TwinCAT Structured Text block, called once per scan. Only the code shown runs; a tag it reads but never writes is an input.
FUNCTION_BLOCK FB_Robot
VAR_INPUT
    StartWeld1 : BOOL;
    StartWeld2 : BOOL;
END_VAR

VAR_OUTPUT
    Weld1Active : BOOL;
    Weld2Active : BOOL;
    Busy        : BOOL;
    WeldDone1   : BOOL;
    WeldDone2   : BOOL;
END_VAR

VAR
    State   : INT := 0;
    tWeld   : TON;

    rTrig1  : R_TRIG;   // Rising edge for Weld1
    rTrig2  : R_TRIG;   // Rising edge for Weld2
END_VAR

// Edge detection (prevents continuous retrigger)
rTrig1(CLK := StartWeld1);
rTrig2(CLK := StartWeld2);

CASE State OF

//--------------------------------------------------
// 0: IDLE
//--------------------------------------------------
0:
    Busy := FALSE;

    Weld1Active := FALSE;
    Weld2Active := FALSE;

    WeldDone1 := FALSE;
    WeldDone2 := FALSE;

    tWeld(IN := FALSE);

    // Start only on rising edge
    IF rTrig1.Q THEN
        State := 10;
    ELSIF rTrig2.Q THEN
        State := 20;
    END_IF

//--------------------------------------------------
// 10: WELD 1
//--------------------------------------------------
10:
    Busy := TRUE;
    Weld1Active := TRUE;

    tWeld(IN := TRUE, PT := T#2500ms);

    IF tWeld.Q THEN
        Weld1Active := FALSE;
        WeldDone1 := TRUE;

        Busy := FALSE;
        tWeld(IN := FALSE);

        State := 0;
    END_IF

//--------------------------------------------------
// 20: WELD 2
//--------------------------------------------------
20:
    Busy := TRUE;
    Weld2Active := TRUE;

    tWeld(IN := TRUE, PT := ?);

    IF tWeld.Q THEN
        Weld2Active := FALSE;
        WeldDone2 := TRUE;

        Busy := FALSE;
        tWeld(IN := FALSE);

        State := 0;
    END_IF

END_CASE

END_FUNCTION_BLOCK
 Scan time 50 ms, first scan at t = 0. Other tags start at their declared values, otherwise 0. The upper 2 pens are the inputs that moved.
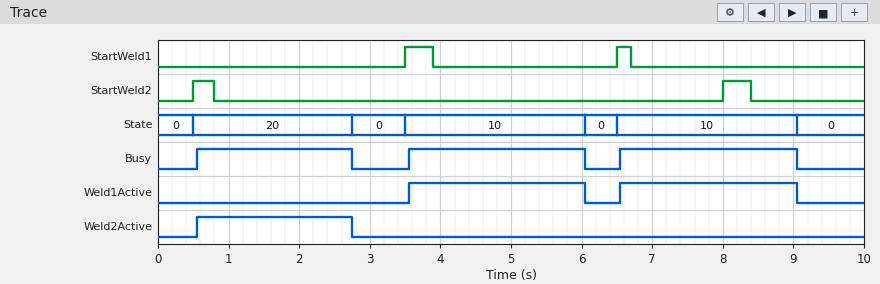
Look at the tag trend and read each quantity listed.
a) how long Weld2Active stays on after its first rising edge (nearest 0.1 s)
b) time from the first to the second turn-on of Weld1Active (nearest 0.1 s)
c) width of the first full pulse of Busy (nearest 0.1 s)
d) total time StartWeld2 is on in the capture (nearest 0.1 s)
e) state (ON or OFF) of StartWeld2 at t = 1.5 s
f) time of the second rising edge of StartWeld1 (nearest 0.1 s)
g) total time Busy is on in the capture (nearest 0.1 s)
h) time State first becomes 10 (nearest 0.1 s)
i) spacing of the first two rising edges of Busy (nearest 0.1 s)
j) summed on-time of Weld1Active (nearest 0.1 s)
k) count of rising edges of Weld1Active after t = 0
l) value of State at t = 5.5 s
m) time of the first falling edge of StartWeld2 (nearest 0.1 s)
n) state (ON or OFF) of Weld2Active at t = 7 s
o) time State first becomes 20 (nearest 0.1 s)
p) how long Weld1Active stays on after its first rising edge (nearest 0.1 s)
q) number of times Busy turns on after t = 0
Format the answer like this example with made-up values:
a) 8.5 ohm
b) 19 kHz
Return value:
a) 2.2 s
b) 3.0 s
c) 2.2 s
d) 0.7 s
e) OFF
f) 6.5 s
g) 7.2 s
h) 3.5 s
i) 3.0 s
j) 5.0 s
k) 2
l) 10
m) 0.8 s
n) OFF
o) 0.5 s
p) 2.5 s
q) 3
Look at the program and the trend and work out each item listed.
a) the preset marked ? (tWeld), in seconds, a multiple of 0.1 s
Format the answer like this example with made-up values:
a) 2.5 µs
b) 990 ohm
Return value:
a) 2.2 s
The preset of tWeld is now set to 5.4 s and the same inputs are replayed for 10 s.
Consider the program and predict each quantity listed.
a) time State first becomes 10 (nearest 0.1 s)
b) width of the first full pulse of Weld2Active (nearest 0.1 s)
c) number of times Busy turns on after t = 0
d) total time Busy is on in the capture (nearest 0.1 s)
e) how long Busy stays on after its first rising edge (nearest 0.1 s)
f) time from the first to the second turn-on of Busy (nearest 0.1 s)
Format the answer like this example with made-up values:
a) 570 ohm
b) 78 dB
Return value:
a) 6.5 s
b) 5.4 s
c) 2
d) 7.9 s
e) 5.4 s
f) 6.0 s
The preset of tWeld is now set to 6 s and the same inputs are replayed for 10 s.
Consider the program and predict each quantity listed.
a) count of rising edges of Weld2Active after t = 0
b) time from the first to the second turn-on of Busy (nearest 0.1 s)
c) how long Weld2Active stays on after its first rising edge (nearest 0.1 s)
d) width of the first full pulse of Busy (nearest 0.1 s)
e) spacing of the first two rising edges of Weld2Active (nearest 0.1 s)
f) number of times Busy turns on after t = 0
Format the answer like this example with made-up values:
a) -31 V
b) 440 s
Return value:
a) 2
b) 7.5 s
c) 6.0 s
d) 6.0 s
e) 7.5 s
f) 2
